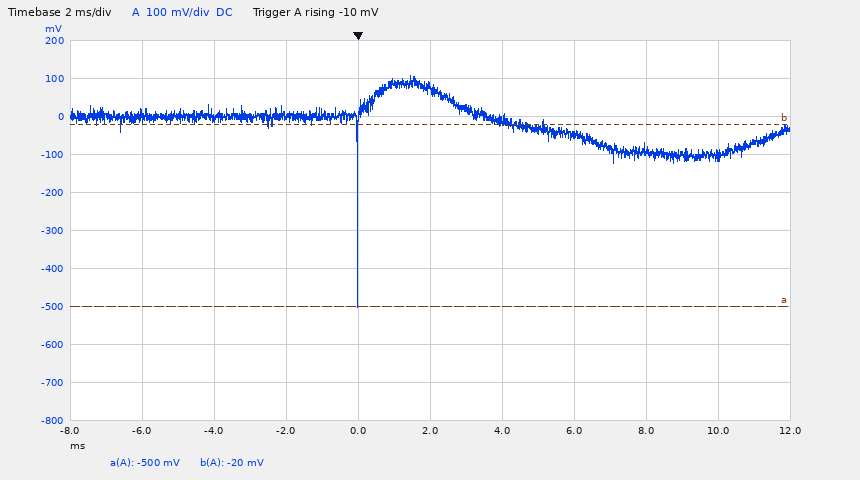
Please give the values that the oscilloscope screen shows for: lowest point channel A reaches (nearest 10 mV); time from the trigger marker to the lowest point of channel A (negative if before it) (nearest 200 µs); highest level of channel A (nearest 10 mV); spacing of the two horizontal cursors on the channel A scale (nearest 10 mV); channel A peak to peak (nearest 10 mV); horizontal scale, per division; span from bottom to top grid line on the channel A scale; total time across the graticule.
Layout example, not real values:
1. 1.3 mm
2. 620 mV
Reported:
1. -500 mV
2. 0.0 ms
3. 110 mV
4. 480 mV
5. 610 mV
6. 2 ms
7. 1 V
8. 20 ms
